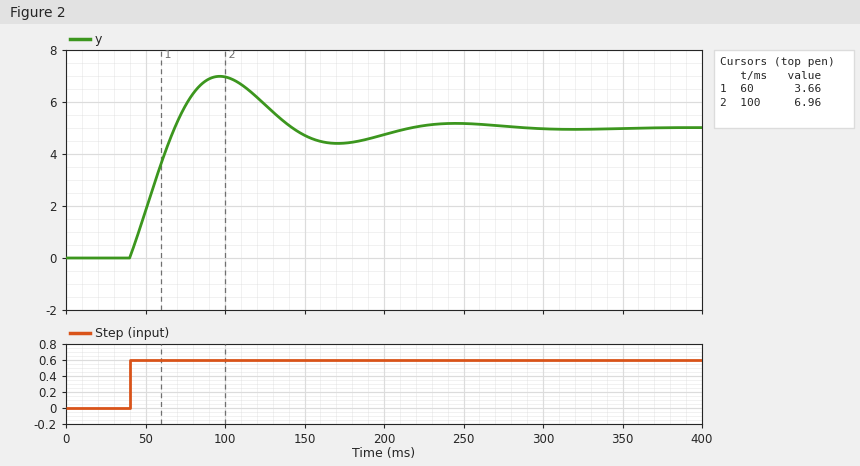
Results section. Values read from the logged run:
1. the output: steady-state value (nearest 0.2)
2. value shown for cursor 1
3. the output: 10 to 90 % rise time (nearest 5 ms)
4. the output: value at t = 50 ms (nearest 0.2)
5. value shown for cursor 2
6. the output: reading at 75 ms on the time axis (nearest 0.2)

5.0
3.66
20 ms
1.8
6.96
5.8
